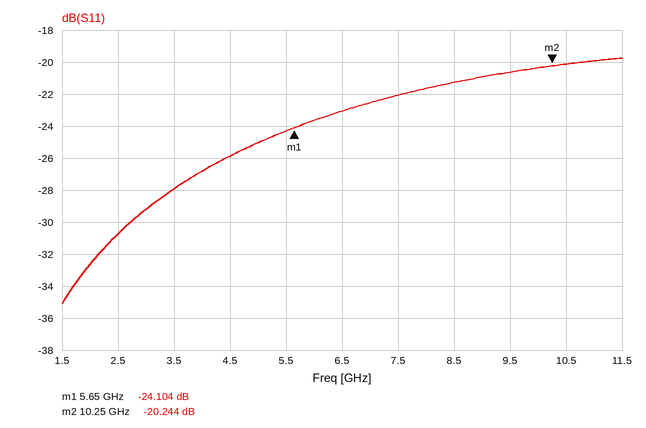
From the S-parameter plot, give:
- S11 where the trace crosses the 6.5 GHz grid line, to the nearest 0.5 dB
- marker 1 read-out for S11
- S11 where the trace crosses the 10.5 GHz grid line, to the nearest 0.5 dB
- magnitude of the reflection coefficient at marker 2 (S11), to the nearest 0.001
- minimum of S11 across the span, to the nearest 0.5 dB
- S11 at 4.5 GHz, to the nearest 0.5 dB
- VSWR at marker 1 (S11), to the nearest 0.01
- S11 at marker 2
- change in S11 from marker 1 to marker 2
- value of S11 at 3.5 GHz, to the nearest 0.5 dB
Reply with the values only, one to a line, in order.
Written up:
-23.0 dB
-24.104 dB
-20.0 dB
0.097
-35.0 dB
-26.0 dB
1.13
-20.244 dB
3.860 dB
-28.0 dB
